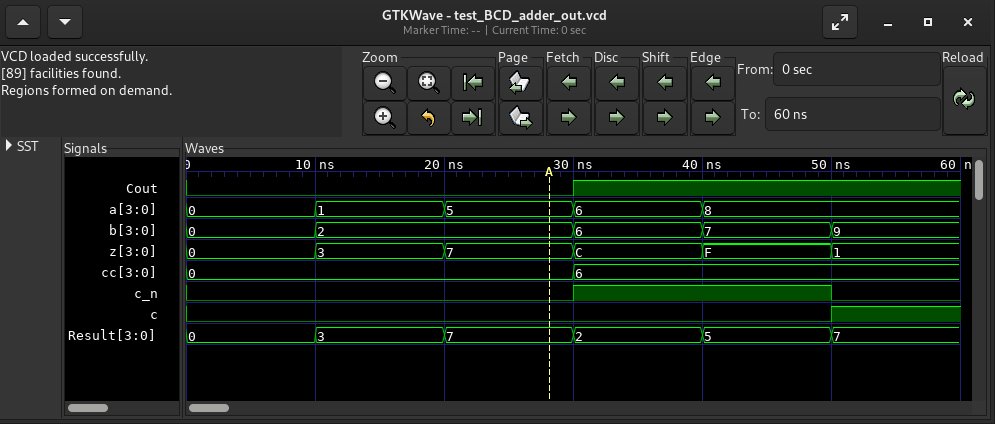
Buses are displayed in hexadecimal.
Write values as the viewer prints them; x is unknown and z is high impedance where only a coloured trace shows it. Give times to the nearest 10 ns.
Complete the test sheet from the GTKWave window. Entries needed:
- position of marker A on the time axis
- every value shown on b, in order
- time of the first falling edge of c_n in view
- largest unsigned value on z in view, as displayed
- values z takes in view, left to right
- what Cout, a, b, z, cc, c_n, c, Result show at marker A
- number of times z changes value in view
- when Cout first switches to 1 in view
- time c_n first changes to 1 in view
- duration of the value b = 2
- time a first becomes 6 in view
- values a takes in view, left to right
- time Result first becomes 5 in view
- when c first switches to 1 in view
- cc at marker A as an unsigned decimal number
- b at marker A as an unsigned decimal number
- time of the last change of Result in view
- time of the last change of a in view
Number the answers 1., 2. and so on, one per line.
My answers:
1. 30 ns
2. 0, 2, 6, 7, 9
3. 50 ns
4. F
5. 0, 3, 7, C, F, 1
6. Cout=0, a=5, b=2, z=7, cc=0, c_n=0, c=0, Result=7
7. 5
8. 30 ns
9. 30 ns
10. 20 ns
11. 30 ns
12. 0, 1, 5, 6, 8
13. 40 ns
14. 50 ns
15. 0
16. 2
17. 50 ns
18. 40 ns
